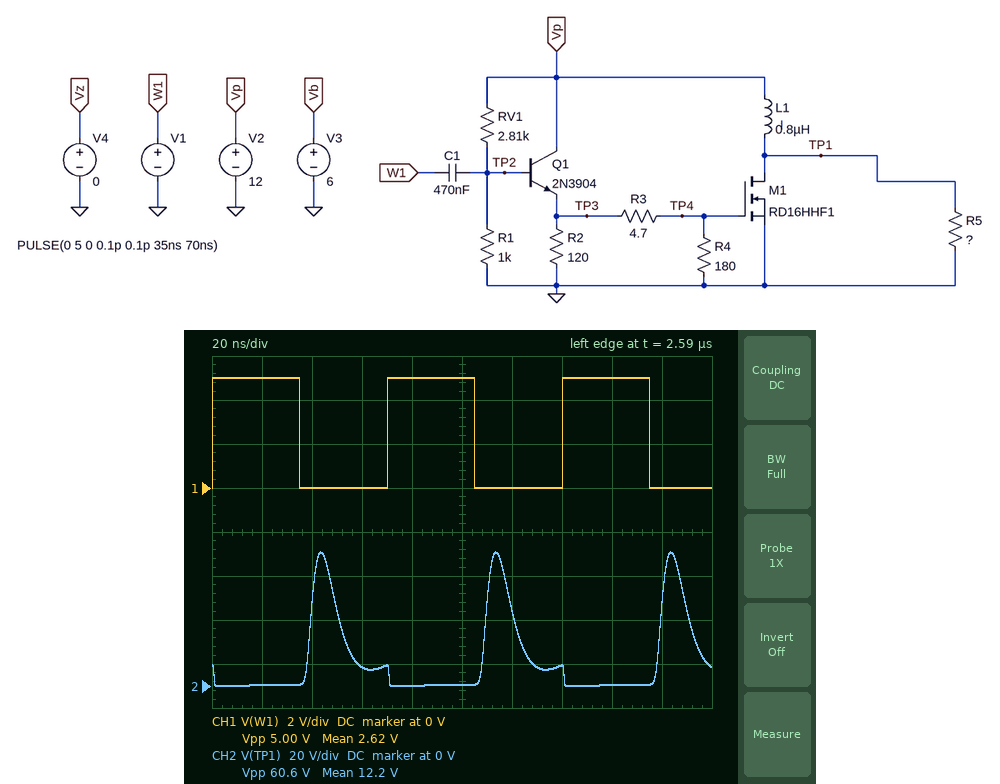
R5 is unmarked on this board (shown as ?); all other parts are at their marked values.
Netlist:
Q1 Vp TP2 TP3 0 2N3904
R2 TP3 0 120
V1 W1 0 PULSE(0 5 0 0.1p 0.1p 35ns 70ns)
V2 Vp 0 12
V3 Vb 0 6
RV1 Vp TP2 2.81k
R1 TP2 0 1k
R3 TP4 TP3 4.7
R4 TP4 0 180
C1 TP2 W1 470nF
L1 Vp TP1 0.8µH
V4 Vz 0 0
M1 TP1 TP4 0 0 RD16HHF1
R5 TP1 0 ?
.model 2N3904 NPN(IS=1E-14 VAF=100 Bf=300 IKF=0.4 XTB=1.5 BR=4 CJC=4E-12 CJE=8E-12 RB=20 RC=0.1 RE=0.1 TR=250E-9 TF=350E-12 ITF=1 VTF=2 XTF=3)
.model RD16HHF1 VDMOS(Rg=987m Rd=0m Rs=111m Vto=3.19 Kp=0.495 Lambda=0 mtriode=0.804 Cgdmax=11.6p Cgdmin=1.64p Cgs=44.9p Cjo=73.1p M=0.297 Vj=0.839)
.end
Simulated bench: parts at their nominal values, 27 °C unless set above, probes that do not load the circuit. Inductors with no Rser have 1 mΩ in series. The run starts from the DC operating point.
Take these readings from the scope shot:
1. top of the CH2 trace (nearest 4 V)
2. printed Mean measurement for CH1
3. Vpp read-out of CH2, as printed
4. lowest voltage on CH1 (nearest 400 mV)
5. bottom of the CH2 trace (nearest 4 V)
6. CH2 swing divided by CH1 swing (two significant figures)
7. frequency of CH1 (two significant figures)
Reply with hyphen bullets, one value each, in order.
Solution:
- 60 V
- 2.62 V
- 60.6 V
- 0 V
- 0 V
- 12
- 14 MHz
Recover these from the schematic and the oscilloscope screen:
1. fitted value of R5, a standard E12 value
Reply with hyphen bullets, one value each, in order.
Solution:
- 150 Ω
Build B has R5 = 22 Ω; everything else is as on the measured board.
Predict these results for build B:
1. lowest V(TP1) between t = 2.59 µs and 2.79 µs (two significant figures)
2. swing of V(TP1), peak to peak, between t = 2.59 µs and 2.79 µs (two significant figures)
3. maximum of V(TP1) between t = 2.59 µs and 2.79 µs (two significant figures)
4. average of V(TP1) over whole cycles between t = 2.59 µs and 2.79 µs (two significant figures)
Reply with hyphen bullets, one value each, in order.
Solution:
- 620 mV
- 28 V
- 29 V
- 12 V
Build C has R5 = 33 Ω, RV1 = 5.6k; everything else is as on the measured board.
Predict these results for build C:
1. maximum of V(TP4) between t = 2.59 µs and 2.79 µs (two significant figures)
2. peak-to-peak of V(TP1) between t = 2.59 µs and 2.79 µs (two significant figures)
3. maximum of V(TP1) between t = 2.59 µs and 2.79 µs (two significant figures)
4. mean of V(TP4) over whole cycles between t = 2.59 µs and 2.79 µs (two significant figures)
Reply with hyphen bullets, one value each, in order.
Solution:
- 6.3 V
- 30 V
- 31 V
- 3.6 V
